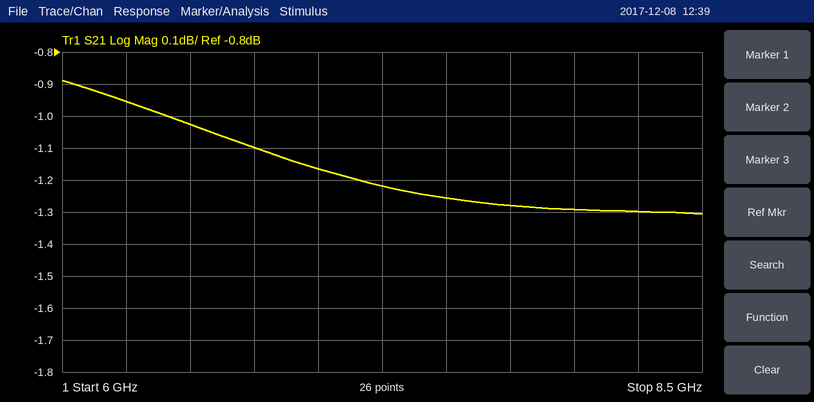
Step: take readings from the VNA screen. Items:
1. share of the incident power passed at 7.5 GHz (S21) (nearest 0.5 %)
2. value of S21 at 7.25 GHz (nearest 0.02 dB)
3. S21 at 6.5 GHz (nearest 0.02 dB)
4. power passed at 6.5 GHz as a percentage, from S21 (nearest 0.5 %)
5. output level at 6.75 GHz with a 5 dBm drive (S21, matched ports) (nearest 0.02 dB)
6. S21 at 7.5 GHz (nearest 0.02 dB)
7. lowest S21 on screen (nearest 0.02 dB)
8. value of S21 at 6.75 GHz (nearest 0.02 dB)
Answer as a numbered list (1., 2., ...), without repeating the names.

1. 75.0 %
2. -1.22 dB
3. -1.02 dB
4. 79.0 %
5. 3.90 dBm
6. -1.26 dB
7. -1.30 dB
8. -1.10 dB
